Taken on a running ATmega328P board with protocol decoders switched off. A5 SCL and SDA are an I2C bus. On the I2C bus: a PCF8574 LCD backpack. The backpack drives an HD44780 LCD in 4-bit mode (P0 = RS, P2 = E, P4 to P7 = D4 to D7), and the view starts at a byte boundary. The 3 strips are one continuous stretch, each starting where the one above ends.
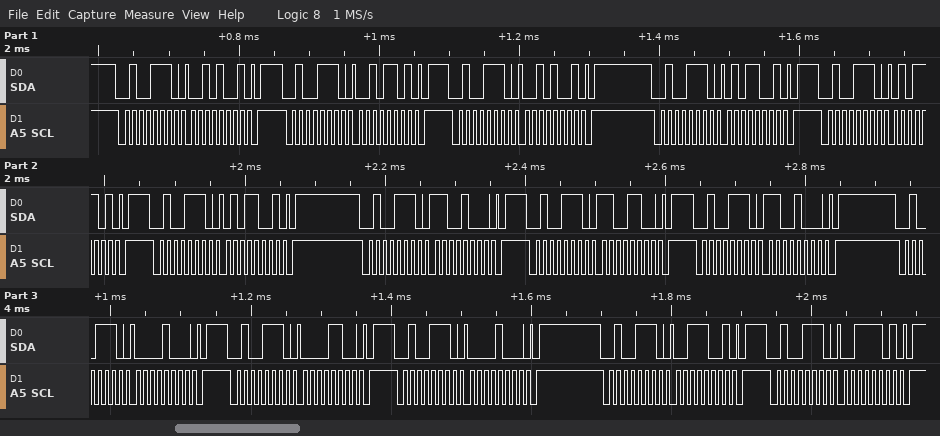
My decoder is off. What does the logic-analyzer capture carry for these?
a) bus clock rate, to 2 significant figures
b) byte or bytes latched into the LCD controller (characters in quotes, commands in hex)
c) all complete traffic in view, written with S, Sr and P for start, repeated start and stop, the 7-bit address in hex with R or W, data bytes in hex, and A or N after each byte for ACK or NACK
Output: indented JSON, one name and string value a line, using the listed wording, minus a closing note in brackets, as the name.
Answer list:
{
  "bus clock rate, to 2 significant figures": "100 kHz",
  "byte or bytes latched into the LCD controller": "'%' 0xC0",
  "all complete traffic in view, written with S, Sr and P for start, repeated start and stop, the 7-bit address in hex with R or W, data bytes in hex, and A or N after each byte for ACK or NACK": "S 27W A 29 A P S 27W A 2D A P S 27W A 29 A P S 27W A 59 A P S 27W A 5D A P S 27W A 59 A P S 27W A C8 A P S 27W A CC A P S 27W A C8 A P S 27W A 08 A P S 27W A 0C A P S 27W A 08 A P S 27W A 39 A P S 27W A 3D A P"
}
